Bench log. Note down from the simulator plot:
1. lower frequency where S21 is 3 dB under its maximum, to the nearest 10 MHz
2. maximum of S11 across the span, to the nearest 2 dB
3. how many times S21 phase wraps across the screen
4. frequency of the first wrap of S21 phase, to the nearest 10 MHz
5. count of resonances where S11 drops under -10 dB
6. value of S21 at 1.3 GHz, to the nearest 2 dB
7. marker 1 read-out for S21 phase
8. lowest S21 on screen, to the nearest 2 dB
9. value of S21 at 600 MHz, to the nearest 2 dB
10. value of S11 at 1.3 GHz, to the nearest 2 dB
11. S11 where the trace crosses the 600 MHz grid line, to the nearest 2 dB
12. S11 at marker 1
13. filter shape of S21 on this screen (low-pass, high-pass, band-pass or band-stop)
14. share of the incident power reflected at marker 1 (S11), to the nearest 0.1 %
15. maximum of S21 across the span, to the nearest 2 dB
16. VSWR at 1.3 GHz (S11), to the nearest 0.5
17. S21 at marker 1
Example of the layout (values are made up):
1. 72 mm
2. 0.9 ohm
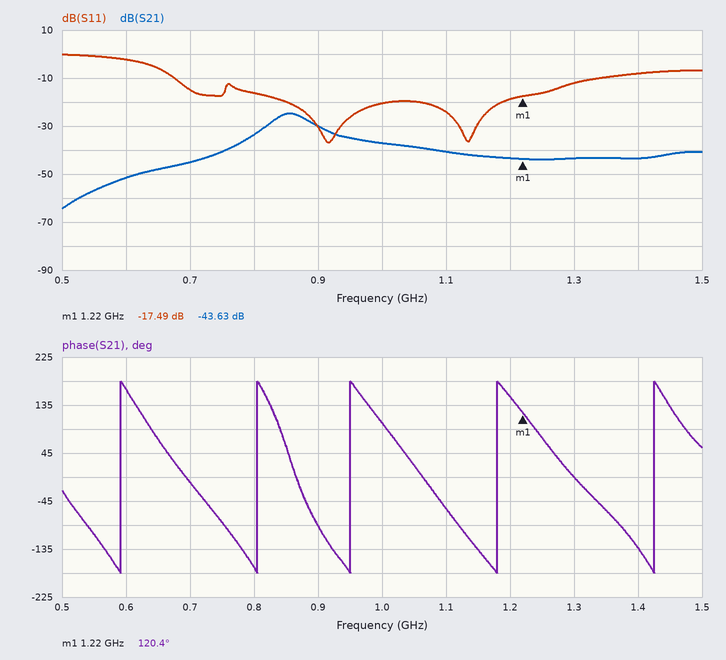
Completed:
1. 830 MHz
2. 0 dB
3. 5
4. 590 MHz
5. 3
6. -44 dB
7. 120.4°
8. -64 dB
9. -52 dB
10. -12 dB
11. -2 dB
12. -17.49 dB
13. band-pass
14. 1.8 %
15. -24 dB
16. 1.5
17. -43.63 dB
